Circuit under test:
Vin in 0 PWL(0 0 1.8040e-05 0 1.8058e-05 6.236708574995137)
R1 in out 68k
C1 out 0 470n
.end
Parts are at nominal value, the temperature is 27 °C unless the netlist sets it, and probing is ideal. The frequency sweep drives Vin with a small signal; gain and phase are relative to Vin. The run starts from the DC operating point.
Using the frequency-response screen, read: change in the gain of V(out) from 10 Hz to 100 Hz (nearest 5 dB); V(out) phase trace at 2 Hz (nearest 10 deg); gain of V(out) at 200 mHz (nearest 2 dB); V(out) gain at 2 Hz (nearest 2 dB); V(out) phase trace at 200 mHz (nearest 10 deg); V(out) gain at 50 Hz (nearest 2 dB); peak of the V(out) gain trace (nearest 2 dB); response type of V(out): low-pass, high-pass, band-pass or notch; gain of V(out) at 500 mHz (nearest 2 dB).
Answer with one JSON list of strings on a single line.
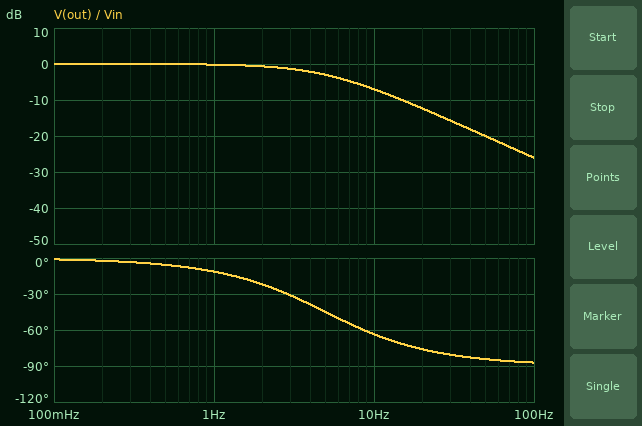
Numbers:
["-20 dB", "-20 deg", "0 dB", "0 dB", "0 deg", "-20 dB", "0 dB", "low-pass", "0 dB"]
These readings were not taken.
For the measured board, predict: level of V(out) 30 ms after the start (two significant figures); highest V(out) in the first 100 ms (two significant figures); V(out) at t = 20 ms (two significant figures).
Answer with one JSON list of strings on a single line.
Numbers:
["3.8 V", "6.0 V", "2.9 V"]
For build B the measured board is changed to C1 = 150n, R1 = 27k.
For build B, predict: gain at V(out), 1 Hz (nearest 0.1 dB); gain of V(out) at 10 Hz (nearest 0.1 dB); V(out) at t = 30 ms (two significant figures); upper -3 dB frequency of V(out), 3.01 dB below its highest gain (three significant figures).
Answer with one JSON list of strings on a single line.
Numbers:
["0 dB", "-0.3 dB", "6.2 V", "39.3 Hz"]
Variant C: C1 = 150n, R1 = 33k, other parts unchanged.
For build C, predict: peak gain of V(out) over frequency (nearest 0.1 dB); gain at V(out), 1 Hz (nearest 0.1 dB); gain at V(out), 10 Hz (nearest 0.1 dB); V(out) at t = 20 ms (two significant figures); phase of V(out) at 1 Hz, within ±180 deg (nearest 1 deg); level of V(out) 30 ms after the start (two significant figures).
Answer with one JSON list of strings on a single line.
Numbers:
["0 dB", "0 dB", "-0.4 dB", "6.1 V", "-2 deg", "6.2 V"]
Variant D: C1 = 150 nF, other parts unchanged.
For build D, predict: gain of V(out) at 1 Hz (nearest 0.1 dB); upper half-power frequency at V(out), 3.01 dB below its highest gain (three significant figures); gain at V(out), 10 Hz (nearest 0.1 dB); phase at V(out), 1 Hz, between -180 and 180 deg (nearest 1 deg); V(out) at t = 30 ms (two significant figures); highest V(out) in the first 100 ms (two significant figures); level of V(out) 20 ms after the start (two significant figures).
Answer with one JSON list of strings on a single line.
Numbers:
["0 dB", "15.6 Hz", "-1.5 dB", "-4 deg", "5.9 V", "6.2 V", "5.4 V"]
